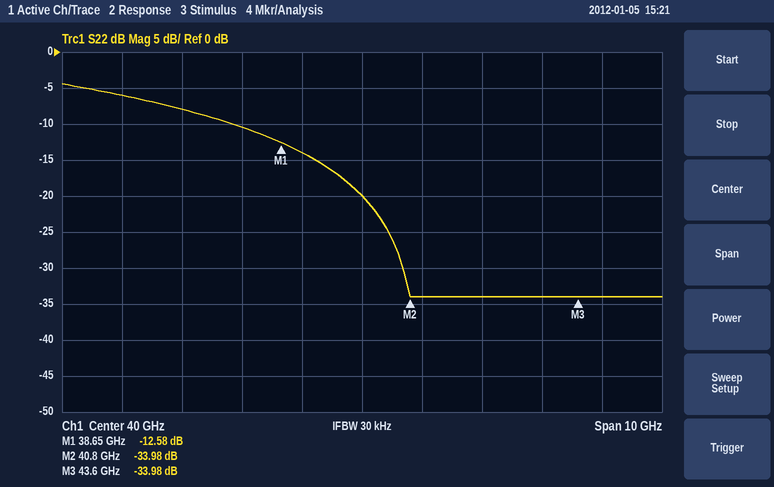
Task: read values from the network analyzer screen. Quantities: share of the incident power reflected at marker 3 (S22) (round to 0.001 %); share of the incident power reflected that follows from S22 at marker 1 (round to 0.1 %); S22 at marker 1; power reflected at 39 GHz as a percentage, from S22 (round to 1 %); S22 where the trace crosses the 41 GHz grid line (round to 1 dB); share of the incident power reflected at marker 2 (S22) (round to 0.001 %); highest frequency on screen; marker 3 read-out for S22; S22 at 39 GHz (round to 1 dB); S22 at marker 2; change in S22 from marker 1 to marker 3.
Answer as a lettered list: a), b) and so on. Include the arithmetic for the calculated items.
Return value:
a) 10^(-33.98/10) ≈ 0.040 %
b) 10^(-12.58/10) ≈ 5.5 %
c) -12.58 dB
d) 10^(-14/10) ≈ 4 %
e) -34 dB
f) 10^(-33.98/10) ≈ 0.040 %
g) 45 GHz
h) -33.98 dB
i) -14 dB
j) -33.98 dB
k) -33.98 − (-12.58) = -21.40 dB
